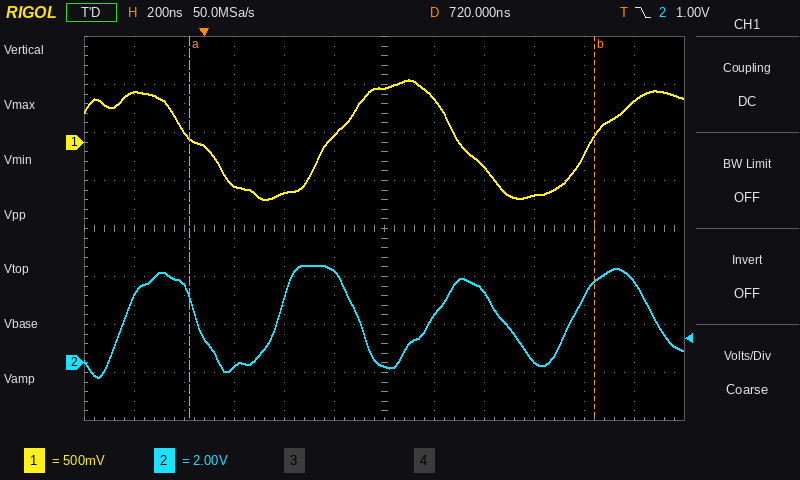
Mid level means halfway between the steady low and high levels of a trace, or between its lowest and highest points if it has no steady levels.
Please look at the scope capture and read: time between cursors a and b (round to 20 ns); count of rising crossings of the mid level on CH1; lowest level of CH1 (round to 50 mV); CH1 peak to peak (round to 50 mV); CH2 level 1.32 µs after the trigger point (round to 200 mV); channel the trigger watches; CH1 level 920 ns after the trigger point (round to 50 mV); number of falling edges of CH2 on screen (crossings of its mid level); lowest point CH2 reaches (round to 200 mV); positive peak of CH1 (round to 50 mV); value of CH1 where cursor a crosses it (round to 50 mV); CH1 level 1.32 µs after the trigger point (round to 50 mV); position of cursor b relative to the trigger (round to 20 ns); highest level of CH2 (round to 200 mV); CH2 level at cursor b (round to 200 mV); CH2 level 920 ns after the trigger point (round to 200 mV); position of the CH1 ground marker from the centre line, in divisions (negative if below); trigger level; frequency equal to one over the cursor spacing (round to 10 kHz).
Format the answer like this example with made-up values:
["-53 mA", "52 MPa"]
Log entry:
["1.62 µs", "2", "-600 mV", "1.25 V", "0.0 V", "CH2", "450 mV", "4", "-600 mV", "650 mV", "50 mV", "-550 mV", "+1.56 µs", "4.0 V", "3.4 V", "2.0 V", "+1.8 div", "1.00 V", "620 kHz"]
